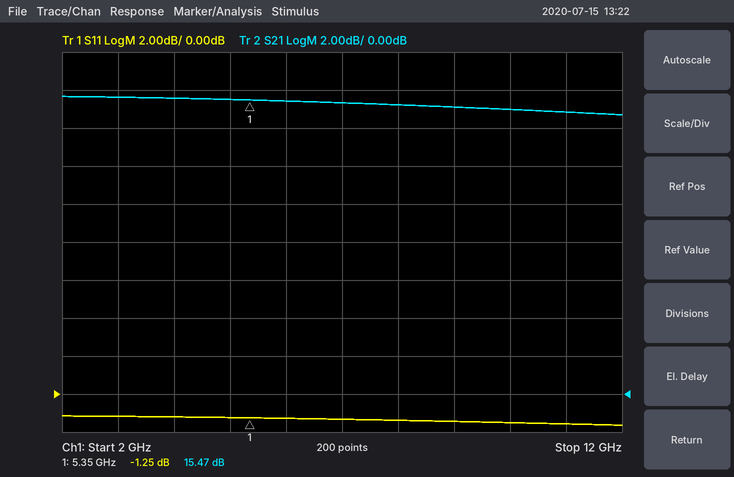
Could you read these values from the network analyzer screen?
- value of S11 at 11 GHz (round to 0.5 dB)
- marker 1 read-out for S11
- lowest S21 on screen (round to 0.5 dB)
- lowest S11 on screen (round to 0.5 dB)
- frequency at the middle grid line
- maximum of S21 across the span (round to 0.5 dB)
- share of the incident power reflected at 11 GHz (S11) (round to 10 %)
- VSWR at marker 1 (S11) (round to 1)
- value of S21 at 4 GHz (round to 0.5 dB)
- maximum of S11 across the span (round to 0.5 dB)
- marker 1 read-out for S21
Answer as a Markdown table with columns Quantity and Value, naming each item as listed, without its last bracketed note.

| Quantity | Value |
|---|---|
| value of S11 at 11 GHz | -1.5 dB |
| marker 1 read-out for S11 | -1.25 dB |
| lowest S21 on screen | 14.5 dB |
| lowest S11 on screen | -1.5 dB |
| frequency at the middle grid line | 7 GHz |
| maximum of S21 across the span | 15.5 dB |
| share of the incident power reflected at 11 GHz (S11) | 70 % |
| VSWR at marker 1 (S11) | 14 |
| value of S21 at 4 GHz | 15.5 dB |
| maximum of S11 across the span | -1.0 dB |
| marker 1 read-out for S21 | 15.47 dB |
